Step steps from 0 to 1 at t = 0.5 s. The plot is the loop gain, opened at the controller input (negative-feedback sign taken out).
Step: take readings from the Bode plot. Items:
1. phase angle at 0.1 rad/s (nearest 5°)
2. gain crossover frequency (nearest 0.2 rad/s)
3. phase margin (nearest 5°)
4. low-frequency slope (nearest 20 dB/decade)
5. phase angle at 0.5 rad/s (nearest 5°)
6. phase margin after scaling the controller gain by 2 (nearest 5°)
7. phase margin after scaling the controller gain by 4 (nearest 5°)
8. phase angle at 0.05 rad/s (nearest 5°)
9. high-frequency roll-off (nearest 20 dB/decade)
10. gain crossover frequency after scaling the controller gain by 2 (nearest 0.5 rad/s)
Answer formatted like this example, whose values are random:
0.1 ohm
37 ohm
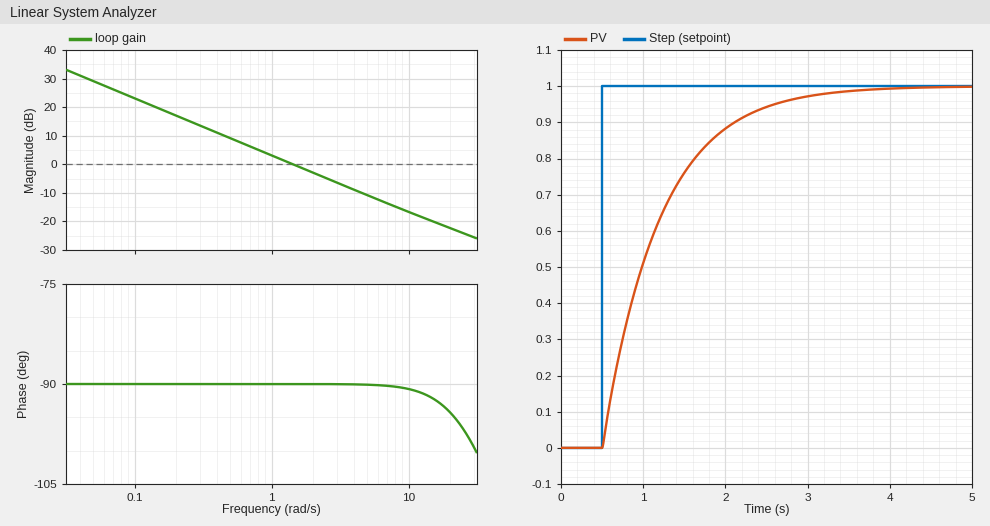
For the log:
-90°
1.4 rad/s
90°
-20 dB/decade
-90°
90°
90°
-90°
-20 dB/decade
3.0 rad/s
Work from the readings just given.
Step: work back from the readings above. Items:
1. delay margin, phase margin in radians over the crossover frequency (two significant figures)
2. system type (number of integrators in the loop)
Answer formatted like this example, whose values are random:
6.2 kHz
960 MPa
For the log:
1.1 s
1
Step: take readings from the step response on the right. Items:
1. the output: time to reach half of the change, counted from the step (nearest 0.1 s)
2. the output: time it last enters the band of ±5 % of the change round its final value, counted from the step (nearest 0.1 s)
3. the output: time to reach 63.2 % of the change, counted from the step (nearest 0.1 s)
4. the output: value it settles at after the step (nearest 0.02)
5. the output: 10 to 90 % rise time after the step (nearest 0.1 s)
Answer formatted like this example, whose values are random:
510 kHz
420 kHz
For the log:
0.5 s
2.1 s
0.7 s
1.00
1.5 s
